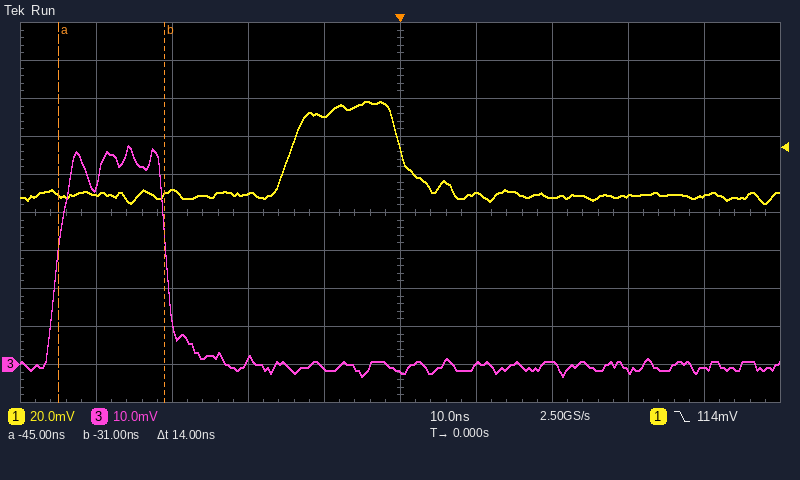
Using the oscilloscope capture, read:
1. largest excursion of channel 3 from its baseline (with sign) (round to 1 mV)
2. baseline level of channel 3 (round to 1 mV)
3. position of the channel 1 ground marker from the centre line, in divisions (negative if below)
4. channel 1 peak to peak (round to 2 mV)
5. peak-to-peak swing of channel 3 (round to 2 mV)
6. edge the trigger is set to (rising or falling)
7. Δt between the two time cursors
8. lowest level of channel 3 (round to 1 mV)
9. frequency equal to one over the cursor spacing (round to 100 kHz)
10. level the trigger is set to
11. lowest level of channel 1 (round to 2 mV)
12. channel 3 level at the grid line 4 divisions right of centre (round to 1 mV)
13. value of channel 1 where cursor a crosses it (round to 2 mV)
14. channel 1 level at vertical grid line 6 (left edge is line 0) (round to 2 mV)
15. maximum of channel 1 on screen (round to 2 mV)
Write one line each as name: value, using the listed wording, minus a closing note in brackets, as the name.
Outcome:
largest excursion of channel 3 from its baseline (with sign): +58 mV
baseline level of channel 3: 0 mV
position of the channel 1 ground marker from the centre line, in divisions: -4.0 div
channel 1 peak to peak: 54 mV
peak-to-peak swing of channel 3: 60 mV
edge the trigger is set to: falling
Δt between the two time cursors: 14 ns
lowest level of channel 3: -3 mV
frequency equal to one over the cursor spacing: 71.4 MHz
level the trigger is set to: 114 mV
lowest level of channel 1: 84 mV
channel 3 level at the grid line 4 divisions right of centre: -1 mV
value of channel 1 where cursor a crosses it: 90 mV
channel 1 level at vertical grid line 6 (left edge is line 0): 90 mV
maximum of channel 1 on screen: 138 mV
